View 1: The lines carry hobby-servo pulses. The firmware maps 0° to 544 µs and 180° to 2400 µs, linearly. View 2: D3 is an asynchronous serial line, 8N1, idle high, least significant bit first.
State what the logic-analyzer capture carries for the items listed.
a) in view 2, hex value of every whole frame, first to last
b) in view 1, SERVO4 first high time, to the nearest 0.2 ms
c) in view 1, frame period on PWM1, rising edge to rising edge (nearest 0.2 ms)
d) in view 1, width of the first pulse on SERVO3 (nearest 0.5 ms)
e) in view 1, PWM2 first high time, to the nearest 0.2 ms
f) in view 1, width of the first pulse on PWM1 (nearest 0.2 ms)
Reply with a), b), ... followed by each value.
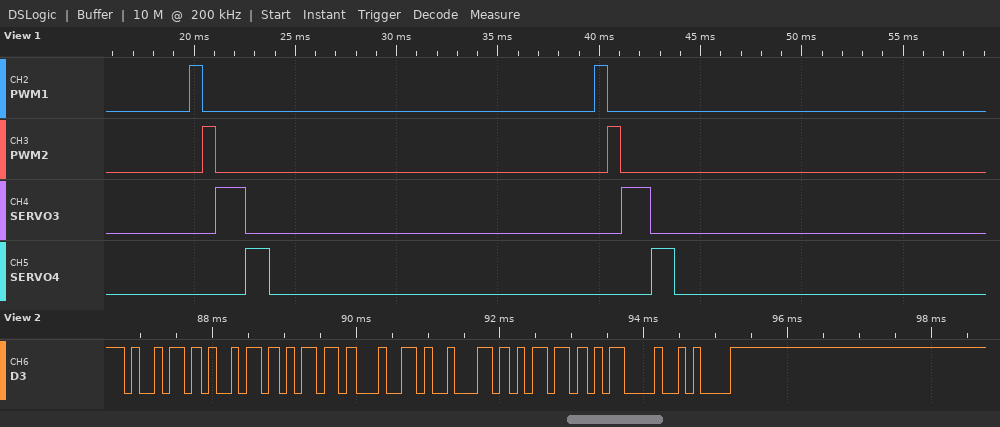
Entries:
a) 69 69 6D 64 62 6D 0D 0A
b) 1.2 ms
c) 20.0 ms
d) 1.5 ms
e) 0.6 ms
f) 0.6 ms
